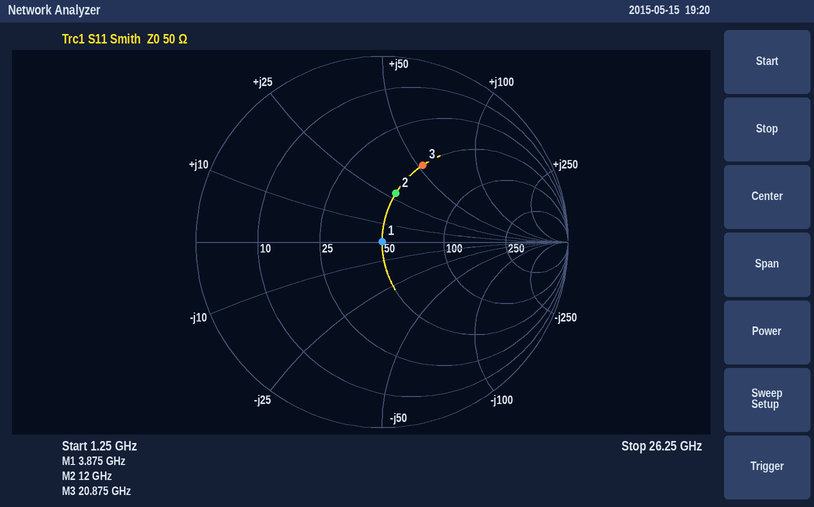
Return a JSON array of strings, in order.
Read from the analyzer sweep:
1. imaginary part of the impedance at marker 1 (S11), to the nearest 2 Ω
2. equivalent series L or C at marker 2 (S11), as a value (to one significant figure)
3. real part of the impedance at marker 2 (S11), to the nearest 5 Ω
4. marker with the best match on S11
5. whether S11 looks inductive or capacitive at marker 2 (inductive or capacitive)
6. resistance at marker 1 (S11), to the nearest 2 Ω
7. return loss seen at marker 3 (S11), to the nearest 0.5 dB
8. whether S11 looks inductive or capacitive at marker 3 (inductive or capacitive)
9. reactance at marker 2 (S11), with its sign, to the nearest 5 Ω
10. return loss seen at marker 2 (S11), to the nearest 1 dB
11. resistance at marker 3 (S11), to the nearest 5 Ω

["0 Ω", "400 pH", "50 Ω", "marker 1", "inductive", "50 Ω", "6.5 dB", "inductive", "+30 Ω", "11 dB", "50 Ω"]
